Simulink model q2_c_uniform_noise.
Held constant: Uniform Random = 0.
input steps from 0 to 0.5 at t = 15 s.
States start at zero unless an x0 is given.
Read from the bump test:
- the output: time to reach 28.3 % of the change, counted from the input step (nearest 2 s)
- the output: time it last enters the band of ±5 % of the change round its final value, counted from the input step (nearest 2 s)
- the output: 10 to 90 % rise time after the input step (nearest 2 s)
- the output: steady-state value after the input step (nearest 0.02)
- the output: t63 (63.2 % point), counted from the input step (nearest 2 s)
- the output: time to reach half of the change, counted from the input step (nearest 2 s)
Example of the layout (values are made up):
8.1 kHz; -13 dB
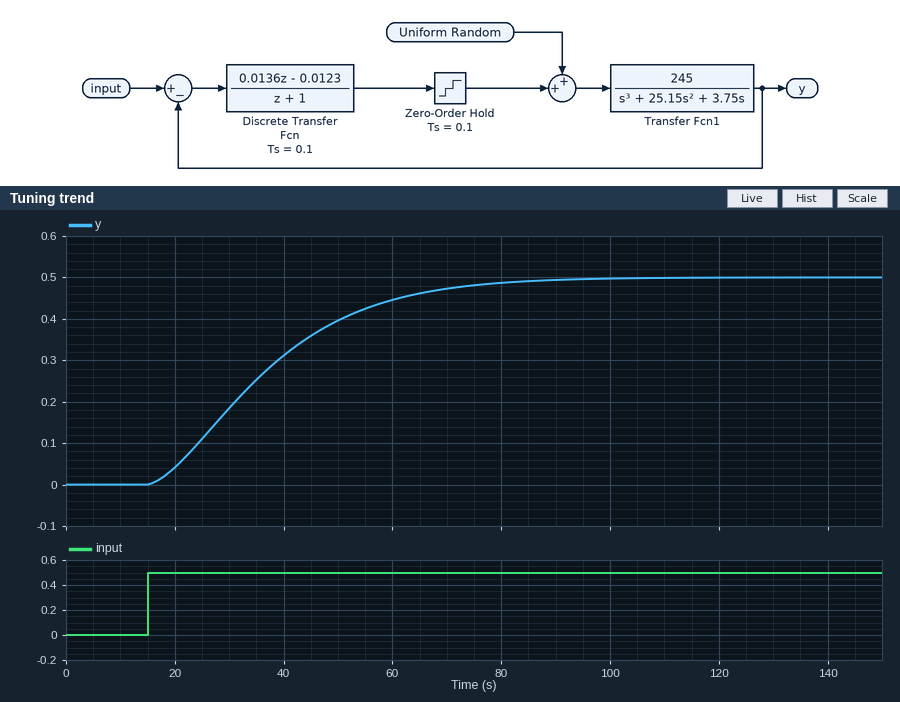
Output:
12 s; 56 s; 40 s; 0.50; 26 s; 20 s
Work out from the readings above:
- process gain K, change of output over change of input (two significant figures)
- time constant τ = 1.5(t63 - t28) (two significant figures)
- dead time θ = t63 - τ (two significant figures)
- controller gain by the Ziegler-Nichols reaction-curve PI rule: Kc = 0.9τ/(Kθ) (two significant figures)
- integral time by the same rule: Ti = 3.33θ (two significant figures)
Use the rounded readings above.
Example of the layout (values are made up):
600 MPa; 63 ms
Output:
1.0; 21 s; 5.0 s; 3.8; 17 s
